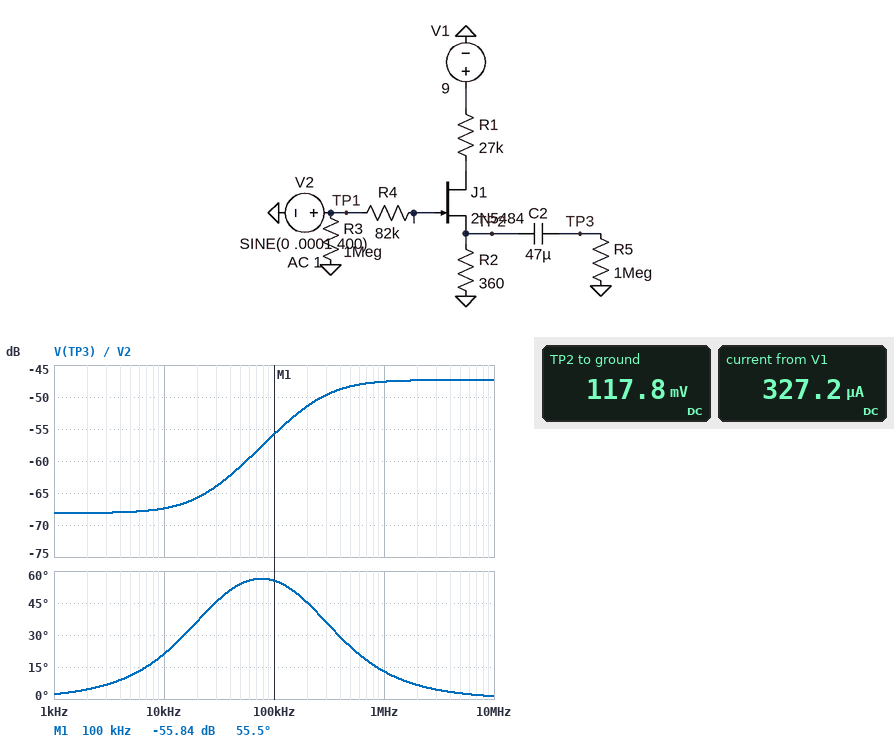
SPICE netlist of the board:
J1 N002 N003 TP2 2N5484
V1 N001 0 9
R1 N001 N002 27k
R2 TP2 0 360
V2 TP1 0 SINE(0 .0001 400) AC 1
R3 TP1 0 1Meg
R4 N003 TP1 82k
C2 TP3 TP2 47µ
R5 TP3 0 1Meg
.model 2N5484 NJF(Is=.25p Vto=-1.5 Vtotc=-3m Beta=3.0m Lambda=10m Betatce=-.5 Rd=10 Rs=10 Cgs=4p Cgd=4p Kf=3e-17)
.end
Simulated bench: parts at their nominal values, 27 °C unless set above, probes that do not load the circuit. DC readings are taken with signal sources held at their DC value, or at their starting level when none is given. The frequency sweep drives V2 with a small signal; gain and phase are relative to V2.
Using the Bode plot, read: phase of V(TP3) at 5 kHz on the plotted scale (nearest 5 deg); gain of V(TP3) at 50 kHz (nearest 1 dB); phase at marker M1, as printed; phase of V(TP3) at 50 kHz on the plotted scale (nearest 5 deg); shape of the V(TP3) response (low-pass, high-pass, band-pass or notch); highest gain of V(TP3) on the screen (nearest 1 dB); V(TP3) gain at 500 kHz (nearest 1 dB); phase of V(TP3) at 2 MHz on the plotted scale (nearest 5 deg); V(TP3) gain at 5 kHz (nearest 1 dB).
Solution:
10 deg
-61 dB
55.5 deg
55 deg
high-pass
-47 dB
-48 dB
5 deg
-68 dB
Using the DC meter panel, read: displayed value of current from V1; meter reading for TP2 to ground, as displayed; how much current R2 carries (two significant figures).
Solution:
327.2 µA
117.8 mV
330 µA
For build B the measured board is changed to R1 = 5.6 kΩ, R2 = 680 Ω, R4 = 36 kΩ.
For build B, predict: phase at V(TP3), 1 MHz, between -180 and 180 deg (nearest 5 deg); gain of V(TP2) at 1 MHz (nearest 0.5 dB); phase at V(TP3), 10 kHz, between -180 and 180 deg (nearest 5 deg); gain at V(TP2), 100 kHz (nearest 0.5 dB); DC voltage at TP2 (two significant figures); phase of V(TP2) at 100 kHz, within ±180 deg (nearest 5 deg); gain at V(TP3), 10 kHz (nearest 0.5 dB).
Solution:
-70 deg
-15.0 dB
0 deg
-3.5 dB
850 mV
-20 deg
-3.0 dB
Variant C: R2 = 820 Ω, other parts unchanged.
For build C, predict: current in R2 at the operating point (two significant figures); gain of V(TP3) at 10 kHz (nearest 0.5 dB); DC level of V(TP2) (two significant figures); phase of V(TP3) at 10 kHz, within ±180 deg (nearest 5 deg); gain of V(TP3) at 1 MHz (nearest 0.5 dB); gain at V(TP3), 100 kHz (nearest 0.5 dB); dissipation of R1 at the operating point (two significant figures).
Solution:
320 µA
-59.0 dB
260 mV
15 deg
-40.5 dB
-49.0 dB
2.8 mW
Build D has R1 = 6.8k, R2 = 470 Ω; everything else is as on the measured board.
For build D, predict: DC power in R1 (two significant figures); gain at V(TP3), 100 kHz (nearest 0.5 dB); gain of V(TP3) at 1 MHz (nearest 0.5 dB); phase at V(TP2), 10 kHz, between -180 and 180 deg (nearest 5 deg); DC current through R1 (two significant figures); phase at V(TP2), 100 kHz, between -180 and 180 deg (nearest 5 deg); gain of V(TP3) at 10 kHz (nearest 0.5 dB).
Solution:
9.8 mW
-33.5 dB
-42.0 dB
0 deg
1.2 mA
-15 deg
-33.0 dB
